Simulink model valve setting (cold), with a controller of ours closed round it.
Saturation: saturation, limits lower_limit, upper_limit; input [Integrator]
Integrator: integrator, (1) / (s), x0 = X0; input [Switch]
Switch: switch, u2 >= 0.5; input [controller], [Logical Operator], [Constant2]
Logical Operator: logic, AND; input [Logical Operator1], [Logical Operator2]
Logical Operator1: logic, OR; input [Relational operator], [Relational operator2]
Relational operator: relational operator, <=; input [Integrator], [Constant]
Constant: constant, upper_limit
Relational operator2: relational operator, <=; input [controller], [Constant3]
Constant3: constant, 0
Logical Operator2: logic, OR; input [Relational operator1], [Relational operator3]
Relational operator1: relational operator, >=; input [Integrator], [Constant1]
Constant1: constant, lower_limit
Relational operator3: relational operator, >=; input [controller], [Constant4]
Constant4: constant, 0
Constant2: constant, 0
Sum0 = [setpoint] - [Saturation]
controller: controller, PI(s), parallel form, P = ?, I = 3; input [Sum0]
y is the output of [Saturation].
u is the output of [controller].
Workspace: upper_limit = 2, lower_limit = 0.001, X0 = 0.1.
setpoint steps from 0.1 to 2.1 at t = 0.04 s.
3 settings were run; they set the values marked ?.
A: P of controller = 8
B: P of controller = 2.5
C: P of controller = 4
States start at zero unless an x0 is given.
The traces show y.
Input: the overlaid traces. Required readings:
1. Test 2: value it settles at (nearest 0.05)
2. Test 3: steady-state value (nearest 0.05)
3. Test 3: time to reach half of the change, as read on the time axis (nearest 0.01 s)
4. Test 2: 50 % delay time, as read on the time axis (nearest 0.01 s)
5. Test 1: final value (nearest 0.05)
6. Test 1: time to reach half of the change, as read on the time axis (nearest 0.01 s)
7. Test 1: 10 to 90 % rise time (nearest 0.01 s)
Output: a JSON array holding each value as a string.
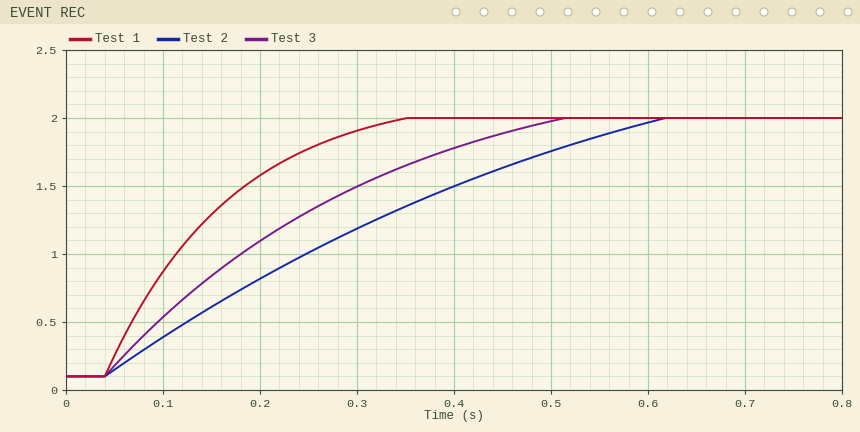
["2.00", "2.00", "0.19 s", "0.26 s", "2.00", "0.12 s", "0.21 s"]
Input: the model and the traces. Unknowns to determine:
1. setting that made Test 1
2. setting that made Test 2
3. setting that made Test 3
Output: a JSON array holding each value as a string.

["A", "B", "C"]
